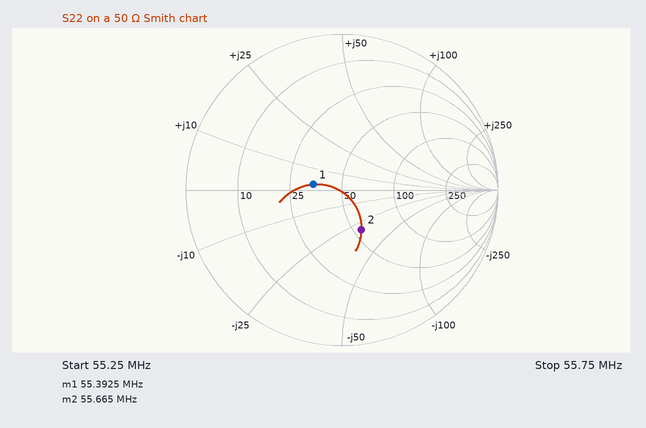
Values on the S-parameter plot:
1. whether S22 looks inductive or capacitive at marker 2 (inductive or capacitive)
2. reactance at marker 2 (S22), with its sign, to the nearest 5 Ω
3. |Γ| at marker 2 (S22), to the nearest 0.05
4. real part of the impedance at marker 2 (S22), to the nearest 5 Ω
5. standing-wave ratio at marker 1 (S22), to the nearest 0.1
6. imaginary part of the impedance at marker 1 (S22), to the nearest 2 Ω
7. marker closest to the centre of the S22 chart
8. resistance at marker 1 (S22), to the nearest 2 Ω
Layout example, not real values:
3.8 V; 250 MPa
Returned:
capacitive; -30 Ω; 0.30; 55 Ω; 1.5; +2 Ω; marker 1; 34 Ω
